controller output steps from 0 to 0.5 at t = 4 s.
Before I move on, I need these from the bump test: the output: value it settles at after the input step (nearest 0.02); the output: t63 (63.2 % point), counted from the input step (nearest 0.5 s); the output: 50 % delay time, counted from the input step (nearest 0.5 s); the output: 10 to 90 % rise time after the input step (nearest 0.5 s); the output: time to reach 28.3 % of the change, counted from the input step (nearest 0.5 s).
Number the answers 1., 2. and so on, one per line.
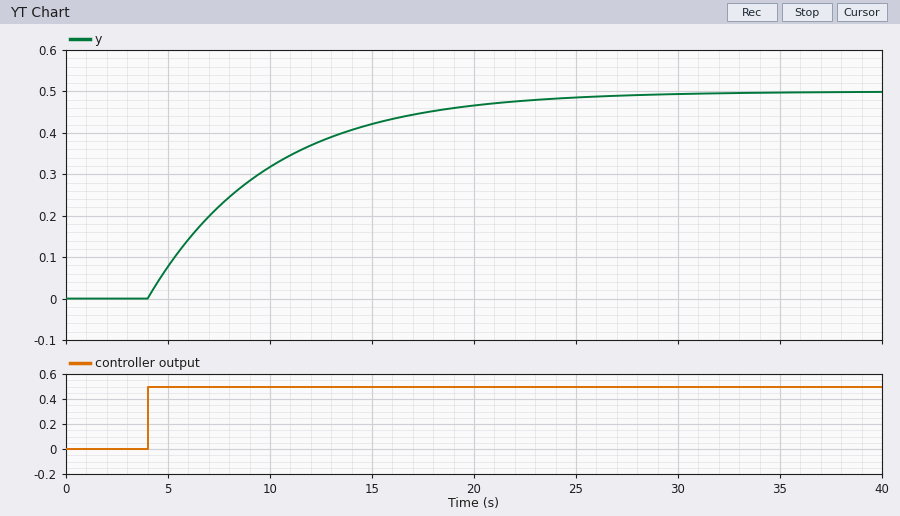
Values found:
1. 0.50
2. 6.0 s
3. 4.0 s
4. 13.0 s
5. 2.0 s
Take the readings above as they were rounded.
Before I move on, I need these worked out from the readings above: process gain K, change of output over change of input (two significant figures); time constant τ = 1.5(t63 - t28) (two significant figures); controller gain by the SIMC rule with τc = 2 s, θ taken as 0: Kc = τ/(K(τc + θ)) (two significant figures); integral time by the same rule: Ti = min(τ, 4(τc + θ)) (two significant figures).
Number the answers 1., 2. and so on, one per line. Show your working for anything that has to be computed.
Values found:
1. (0.5 - 0) / 0.5 = 1.0
2. 1.5 × (6 - 2) = 6.0 s
3. 6 / (1 × (2 + 0)) = 3.0
4. min(6, 4 × (2 + 0)) = 6.0 s
